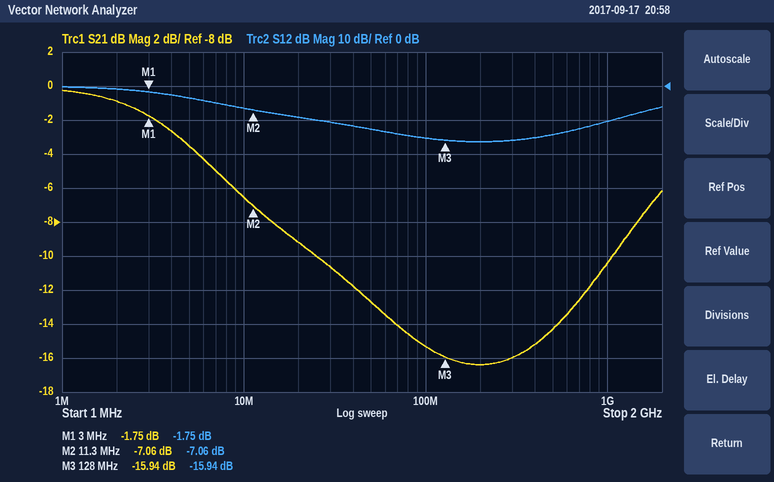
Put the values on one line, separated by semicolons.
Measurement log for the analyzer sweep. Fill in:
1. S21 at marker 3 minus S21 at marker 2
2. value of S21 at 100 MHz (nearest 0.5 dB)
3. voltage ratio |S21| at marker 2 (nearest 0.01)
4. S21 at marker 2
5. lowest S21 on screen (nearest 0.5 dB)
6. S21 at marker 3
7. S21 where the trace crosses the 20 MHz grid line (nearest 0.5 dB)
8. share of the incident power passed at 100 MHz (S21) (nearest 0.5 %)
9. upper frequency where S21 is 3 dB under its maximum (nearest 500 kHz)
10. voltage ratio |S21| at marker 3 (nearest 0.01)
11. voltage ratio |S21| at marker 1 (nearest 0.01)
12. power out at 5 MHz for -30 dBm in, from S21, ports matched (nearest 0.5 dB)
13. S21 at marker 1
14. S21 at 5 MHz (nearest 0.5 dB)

-8.88 dB; -15.5 dB; 0.44; -7.06 dB; -16.5 dB; -15.94 dB; -9.0 dB; 3.0 %; 4.5 MHz; 0.16; 0.82; -33.5 dBm; -1.75 dB; -3.5 dB
